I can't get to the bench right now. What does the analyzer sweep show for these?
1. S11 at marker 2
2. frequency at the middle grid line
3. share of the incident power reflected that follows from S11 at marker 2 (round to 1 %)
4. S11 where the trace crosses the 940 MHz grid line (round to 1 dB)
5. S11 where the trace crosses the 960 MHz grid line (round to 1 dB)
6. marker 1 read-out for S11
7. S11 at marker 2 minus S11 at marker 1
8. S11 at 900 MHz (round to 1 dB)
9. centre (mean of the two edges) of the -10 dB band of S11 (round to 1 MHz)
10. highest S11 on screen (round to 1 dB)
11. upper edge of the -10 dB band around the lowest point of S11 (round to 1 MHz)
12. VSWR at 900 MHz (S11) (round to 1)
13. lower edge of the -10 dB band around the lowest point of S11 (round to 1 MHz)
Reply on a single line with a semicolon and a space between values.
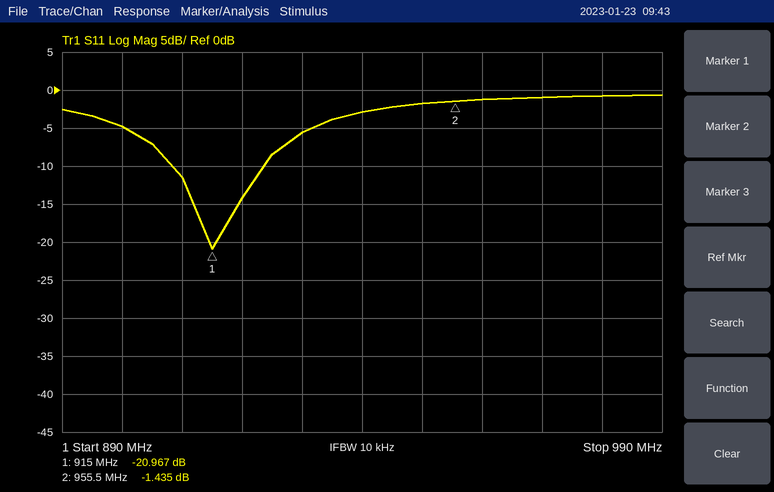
-1.435 dB; 940 MHz; 72 %; -3 dB; -1 dB; -20.967 dB; 19.532 dB; -5 dB; 916 MHz; -1 dB; 924 MHz; 4; 908 MHz
